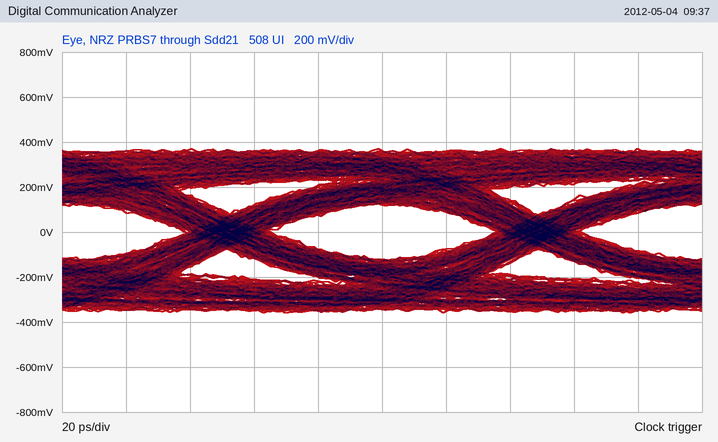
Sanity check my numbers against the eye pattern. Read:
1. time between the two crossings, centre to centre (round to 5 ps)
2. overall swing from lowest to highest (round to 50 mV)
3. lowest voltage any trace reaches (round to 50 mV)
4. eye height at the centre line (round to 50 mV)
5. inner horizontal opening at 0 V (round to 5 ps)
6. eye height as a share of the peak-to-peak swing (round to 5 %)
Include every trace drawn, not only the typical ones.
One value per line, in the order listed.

95 ps
750 mV
-350 mV
250 mV
70 ps
35 %
